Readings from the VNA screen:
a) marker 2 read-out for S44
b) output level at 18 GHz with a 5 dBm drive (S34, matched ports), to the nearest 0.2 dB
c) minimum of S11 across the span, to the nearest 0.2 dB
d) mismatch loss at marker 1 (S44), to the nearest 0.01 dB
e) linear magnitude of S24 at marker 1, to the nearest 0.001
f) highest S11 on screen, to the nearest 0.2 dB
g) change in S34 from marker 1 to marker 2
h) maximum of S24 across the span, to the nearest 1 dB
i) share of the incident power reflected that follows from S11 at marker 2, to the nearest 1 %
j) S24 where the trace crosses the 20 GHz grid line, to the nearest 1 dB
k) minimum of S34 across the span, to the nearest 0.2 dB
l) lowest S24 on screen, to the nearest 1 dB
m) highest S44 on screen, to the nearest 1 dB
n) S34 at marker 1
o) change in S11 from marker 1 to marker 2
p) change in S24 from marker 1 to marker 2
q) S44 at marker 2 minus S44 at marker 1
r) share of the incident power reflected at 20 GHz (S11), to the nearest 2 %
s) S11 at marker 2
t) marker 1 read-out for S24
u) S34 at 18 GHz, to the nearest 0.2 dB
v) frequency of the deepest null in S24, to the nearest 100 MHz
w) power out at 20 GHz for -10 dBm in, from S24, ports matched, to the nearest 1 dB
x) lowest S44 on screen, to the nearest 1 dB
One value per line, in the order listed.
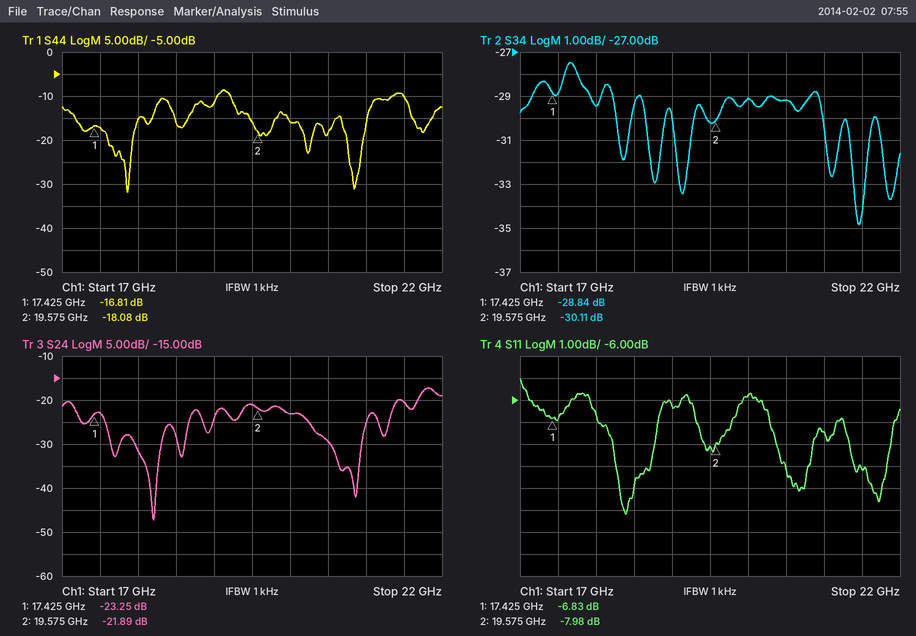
-18.08 dB
-24.4 dBm
-11.2 dB
0.09 dB
0.069
-5.0 dB
-1.27 dB
-17 dB
16 %
-23 dB
-34.8 dB
-47 dB
-9 dB
-28.84 dB
-1.15 dB
1.36 dB
-1.27 dB
26 %
-7.98 dB
-23.25 dB
-29.4 dB
18.2 GHz
-33 dBm
-32 dB
